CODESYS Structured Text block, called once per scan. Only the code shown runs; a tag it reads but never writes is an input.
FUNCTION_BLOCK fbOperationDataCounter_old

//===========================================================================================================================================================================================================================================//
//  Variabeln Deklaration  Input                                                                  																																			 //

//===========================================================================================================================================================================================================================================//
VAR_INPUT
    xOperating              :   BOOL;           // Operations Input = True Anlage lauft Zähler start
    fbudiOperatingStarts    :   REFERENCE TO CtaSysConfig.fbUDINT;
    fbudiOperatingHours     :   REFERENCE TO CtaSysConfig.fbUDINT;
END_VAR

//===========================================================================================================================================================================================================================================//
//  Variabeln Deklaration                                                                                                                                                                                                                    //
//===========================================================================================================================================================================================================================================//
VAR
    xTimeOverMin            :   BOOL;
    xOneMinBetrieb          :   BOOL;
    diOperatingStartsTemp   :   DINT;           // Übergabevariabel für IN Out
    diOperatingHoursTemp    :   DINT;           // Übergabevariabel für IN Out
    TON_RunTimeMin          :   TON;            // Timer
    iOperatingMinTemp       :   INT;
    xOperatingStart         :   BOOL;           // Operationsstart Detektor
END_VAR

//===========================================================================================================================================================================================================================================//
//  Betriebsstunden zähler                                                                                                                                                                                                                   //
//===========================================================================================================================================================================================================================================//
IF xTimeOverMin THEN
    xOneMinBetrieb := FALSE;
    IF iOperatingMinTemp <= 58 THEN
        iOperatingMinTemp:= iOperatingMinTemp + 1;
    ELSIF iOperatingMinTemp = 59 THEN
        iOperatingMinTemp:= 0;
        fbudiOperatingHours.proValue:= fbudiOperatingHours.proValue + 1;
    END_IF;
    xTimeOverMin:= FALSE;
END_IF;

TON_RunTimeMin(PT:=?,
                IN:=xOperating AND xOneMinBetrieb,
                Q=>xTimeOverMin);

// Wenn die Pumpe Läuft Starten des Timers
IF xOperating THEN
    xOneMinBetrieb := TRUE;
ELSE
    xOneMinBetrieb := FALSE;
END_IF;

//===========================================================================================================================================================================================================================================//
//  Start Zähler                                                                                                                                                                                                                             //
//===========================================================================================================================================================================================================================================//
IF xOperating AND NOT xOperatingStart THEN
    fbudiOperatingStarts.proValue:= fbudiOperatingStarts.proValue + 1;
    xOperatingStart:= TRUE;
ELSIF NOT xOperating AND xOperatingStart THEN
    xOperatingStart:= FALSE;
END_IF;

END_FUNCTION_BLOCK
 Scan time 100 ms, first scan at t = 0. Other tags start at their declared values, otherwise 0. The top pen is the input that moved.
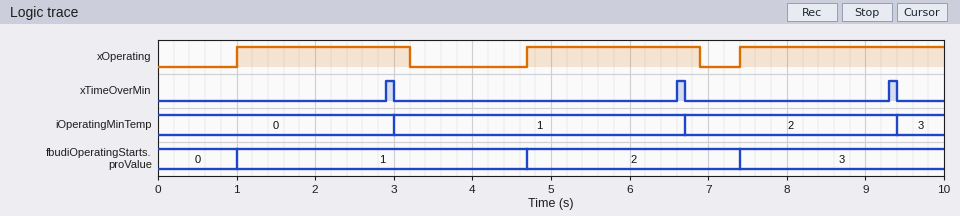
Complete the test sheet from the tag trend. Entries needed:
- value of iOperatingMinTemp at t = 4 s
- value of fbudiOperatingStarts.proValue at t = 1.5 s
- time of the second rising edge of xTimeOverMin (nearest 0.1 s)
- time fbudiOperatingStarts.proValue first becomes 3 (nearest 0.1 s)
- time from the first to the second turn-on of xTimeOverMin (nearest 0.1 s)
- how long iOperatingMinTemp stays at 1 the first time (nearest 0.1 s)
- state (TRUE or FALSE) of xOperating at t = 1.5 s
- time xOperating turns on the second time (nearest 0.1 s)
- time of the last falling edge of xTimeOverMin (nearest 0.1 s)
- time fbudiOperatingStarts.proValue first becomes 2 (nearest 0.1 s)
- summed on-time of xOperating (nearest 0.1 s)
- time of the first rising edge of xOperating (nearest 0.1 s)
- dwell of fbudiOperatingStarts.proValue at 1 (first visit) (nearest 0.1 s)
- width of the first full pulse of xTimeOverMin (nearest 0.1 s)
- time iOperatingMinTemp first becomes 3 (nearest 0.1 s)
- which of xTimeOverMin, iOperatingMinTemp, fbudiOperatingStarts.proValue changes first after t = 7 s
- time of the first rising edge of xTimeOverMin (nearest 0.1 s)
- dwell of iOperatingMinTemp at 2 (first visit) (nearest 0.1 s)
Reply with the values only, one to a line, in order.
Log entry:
1
1
6.6 s
7.4 s
3.7 s
3.7 s
TRUE
4.7 s
9.4 s
4.7 s
7.0 s
1.0 s
3.7 s
0.1 s
9.4 s
fbudiOperatingStarts.proValue
2.9 s
2.7 s
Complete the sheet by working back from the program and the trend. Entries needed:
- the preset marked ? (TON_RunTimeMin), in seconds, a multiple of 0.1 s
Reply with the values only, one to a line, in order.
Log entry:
1.8 s
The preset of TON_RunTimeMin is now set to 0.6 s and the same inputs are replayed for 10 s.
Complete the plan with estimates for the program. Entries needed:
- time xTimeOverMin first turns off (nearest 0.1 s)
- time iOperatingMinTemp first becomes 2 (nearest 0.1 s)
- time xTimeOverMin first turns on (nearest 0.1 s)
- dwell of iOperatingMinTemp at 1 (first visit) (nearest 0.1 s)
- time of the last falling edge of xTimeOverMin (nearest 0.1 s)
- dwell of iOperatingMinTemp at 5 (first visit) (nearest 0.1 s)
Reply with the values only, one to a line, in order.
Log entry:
1.8 s
2.6 s
1.7 s
0.8 s
9.8 s
0.8 s
